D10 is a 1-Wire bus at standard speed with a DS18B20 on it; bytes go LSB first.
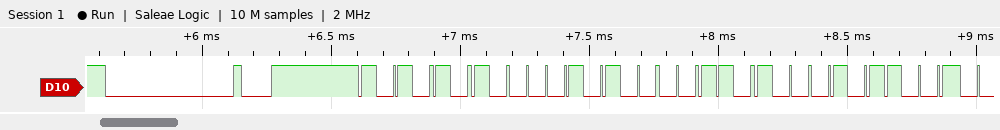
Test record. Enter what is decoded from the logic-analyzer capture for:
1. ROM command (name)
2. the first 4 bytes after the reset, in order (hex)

Match ROM
55 28 2C 9A
